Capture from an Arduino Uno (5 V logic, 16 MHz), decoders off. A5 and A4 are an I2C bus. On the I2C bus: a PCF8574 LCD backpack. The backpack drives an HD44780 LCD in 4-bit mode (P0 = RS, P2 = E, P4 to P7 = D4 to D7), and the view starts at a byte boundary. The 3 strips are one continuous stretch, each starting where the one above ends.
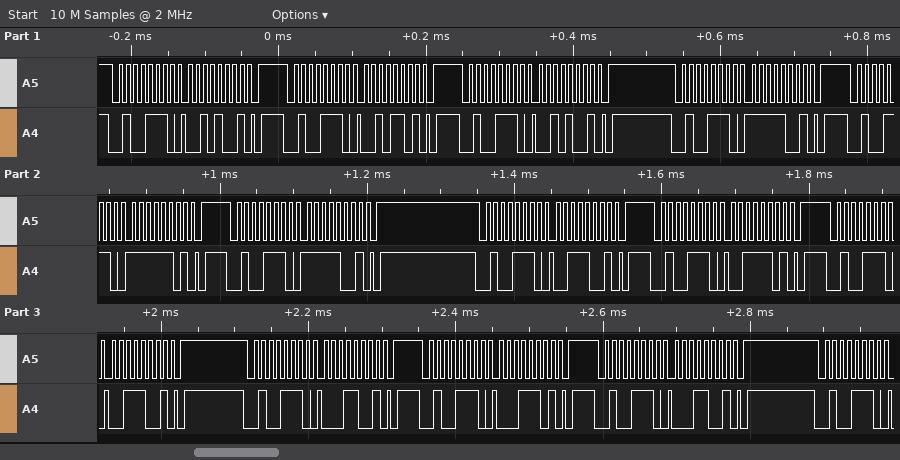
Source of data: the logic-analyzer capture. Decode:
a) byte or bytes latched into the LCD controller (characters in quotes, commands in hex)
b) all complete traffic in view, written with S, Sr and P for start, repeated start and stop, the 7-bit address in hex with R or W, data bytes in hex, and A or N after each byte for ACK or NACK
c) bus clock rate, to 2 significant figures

'/' '1'
S 27W A 29 A P S 27W A 2D A P S 27W A 29 A P S 27W A F9 A P S 27W A FD A P S 27W A F9 A P S 27W A 39 A P S 27W A 3D A P S 27W A 39 A P S 27W A 19 A P S 27W A 1D A P S 27W A 19 A P S 27W A
100 kHz
